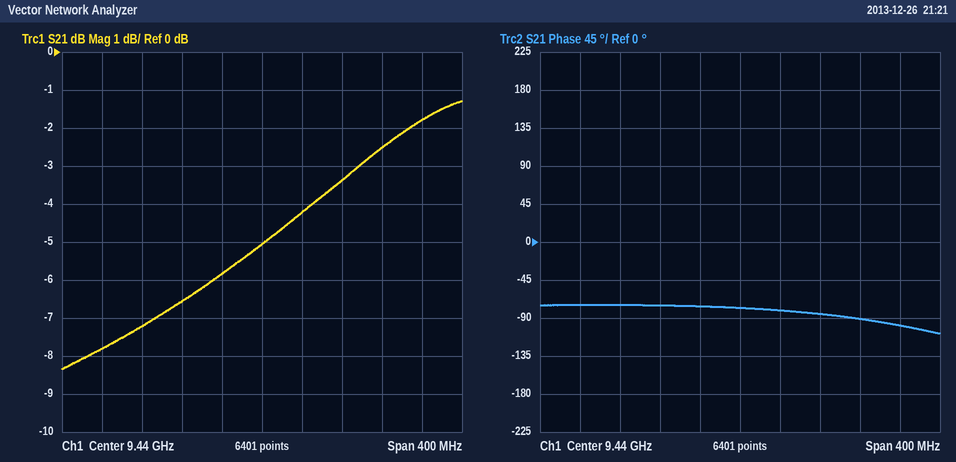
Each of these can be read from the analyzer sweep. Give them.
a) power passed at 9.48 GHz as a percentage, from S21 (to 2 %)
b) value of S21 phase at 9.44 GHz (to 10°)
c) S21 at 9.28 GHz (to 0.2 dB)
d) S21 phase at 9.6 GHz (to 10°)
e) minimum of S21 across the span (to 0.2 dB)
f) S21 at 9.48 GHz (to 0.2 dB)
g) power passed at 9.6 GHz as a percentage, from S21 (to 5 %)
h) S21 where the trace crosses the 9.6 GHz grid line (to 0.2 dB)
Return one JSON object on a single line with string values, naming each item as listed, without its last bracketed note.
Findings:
{"power passed at 9.48 GHz as a percentage, from S21": "38 %", "value of S21 phase at 9.44 GHz": "-80°", "S21 at 9.28 GHz": "-7.8 dB", "S21 phase at 9.6 GHz": "-100°", "minimum of S21 across the span": "-8.4 dB", "S21 at 9.48 GHz": "-4.2 dB", "power passed at 9.6 GHz as a percentage, from S21": "65 %", "S21 where the trace crosses the 9.6 GHz grid line": "-1.8 dB"}
